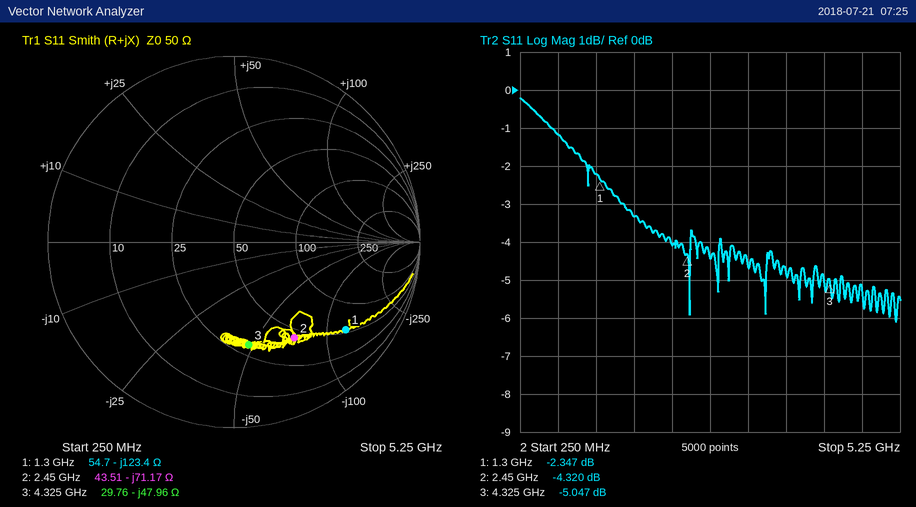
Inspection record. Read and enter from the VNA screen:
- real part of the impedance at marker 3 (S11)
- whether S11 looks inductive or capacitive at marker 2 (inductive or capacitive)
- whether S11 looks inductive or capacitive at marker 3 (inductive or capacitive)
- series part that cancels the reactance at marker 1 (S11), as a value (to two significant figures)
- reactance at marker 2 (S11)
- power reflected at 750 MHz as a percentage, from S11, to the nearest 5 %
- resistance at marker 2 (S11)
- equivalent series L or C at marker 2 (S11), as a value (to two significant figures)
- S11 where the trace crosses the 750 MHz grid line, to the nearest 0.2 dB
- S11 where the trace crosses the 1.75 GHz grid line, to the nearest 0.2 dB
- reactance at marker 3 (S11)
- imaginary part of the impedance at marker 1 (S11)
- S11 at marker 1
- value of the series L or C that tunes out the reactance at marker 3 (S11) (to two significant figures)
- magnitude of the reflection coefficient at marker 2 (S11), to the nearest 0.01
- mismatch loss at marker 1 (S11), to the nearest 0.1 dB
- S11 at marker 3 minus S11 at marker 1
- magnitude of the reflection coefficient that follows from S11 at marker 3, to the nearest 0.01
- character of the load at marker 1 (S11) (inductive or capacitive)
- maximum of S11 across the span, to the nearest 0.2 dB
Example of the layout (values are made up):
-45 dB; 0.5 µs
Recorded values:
29.76 Ω; capacitive; capacitive; 15 nH; -71.17 Ω; 75 %; 43.51 Ω; 910 fF; -1.2 dB; -3.4 dB; -47.96 Ω; -123.4 Ω; -2.347 dB; 1.8 nH; 0.61; 3.8 dB; -2.700 dB; 0.56; capacitive; -0.2 dB
